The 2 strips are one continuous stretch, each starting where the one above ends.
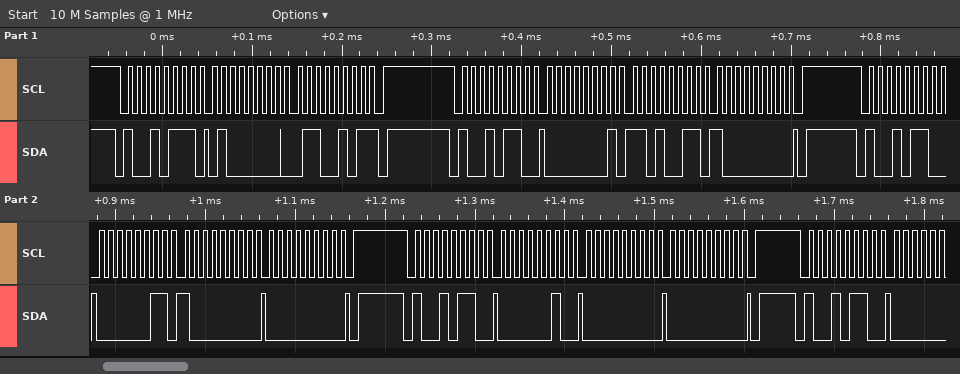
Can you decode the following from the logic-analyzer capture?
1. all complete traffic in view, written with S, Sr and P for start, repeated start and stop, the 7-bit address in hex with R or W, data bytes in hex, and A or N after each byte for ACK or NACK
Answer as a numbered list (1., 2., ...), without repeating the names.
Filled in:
1. S 4BR A 40 A 65 N P S 4BW A 01 A D3 A 80 A P S 4BW A 03 A 80 A 00 A P S 4BW A 02 A 00 A 00 A P S 4BW A
